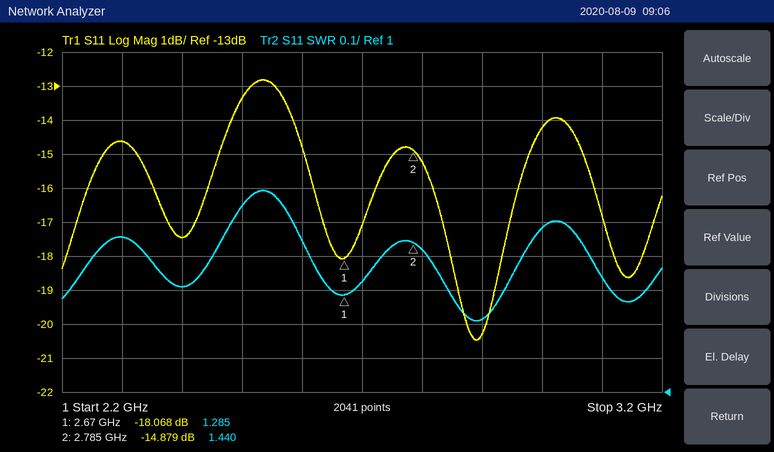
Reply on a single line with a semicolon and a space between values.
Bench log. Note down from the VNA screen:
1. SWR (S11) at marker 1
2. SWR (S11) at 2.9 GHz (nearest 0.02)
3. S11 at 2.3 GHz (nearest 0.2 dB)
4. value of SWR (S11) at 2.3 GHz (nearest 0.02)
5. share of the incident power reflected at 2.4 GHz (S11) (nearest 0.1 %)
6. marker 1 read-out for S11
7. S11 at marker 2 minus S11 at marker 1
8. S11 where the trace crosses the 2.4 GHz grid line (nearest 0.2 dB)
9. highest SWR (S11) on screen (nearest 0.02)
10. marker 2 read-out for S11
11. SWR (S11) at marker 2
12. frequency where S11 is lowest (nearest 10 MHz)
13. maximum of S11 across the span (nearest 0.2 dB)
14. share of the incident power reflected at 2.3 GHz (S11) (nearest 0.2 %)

1.285; 1.22; -14.6 dB; 1.46; 1.8 %; -18.068 dB; 3.189 dB; -17.4 dB; 1.60; -14.879 dB; 1.440; 2.89 GHz; -12.8 dB; 3.4 %
